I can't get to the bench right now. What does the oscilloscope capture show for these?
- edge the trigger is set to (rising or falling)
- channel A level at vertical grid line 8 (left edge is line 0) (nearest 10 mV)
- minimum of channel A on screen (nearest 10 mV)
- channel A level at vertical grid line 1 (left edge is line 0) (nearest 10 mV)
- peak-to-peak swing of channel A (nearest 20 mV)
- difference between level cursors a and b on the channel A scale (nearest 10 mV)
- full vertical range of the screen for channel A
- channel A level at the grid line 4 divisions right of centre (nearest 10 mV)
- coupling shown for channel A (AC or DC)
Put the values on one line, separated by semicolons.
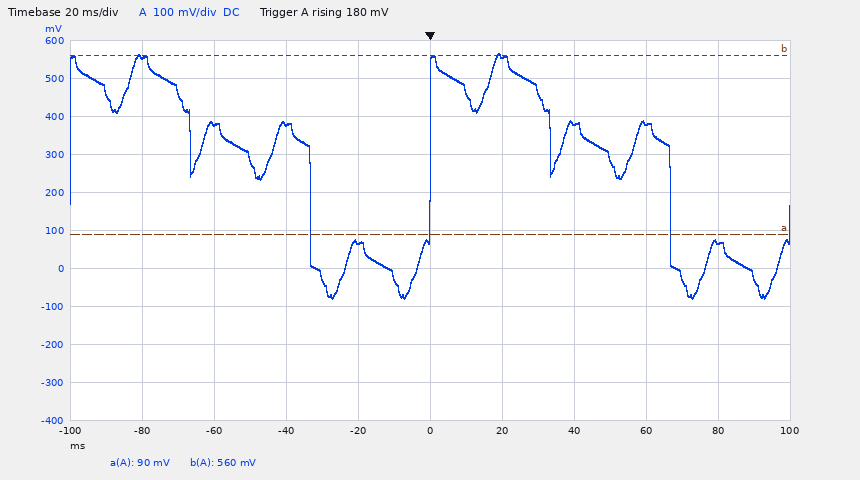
rising; 380 mV; -80 mV; 560 mV; 640 mV; 470 mV; 1 V; 70 mV; DC
